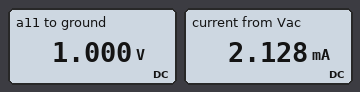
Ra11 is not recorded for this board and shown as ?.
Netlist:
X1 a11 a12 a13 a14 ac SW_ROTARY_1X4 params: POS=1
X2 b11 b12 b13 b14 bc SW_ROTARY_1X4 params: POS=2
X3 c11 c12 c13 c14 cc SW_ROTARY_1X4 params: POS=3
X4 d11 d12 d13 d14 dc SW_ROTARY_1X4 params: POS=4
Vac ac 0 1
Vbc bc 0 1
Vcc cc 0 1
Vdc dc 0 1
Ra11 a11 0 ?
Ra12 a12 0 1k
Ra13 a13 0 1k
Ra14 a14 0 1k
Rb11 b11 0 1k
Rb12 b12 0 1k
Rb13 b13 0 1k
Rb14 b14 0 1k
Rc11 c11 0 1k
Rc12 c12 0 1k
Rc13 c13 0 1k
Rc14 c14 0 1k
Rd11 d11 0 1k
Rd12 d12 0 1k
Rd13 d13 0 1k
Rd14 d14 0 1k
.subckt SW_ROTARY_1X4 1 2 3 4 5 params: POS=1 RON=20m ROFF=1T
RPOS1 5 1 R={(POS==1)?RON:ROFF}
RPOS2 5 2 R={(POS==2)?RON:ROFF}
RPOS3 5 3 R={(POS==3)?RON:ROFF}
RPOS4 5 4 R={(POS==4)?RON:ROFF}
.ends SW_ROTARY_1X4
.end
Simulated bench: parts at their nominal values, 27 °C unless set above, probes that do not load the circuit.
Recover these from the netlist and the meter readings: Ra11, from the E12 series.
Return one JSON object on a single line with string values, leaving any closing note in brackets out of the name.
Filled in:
{"Ra11, from the E12 series": "470 Ω"}
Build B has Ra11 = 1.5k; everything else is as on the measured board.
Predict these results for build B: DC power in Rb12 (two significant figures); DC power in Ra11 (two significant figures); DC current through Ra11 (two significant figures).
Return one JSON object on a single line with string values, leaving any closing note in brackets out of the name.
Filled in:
{"DC power in Rb12": "1.0 mW", "DC power in Ra11": "670 µW", "DC current through Ra11": "670 µA"}
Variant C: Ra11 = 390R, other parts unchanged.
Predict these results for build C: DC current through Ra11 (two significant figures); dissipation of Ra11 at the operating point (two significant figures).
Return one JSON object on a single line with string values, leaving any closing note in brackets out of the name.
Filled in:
{"DC current through Ra11": "2.6 mA", "dissipation of Ra11 at the operating point": "2.6 mW"}
